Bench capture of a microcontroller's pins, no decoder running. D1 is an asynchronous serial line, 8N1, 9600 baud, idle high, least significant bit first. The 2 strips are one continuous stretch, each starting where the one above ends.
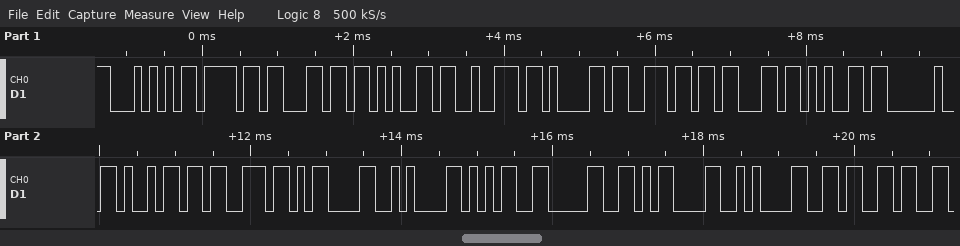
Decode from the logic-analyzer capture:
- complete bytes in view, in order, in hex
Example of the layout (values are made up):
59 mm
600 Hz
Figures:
54 6F 6C 65 72 61 6E 63 65 20 69 73 0D 0A 35 30 0D 0A 36
